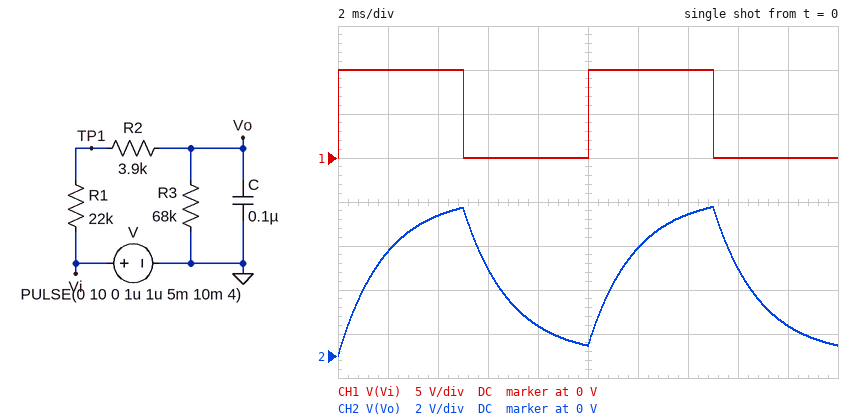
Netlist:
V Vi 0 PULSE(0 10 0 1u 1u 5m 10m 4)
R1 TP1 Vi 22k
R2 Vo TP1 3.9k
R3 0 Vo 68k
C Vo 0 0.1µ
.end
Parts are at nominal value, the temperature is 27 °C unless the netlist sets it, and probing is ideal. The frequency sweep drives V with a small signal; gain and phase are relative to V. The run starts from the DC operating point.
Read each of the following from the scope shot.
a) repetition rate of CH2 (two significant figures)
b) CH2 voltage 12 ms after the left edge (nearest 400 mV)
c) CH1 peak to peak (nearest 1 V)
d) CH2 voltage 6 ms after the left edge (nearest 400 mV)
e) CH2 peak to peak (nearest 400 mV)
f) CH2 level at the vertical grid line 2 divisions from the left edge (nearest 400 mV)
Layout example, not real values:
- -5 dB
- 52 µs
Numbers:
- 100 Hz
- 4.8 V
- 10 V
- 4.0 V
- 6.8 V
- 6.4 V
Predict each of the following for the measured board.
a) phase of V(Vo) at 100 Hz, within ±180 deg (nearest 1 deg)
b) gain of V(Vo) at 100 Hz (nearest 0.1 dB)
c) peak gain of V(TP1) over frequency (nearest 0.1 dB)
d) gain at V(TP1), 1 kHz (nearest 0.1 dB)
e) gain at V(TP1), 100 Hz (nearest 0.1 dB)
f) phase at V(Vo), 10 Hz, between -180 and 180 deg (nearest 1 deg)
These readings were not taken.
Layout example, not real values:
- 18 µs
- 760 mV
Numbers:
- -50 deg
- -6.6 dB
- -2.3 dB
- -15.7 dB
- -5.9 dB
- -7 deg
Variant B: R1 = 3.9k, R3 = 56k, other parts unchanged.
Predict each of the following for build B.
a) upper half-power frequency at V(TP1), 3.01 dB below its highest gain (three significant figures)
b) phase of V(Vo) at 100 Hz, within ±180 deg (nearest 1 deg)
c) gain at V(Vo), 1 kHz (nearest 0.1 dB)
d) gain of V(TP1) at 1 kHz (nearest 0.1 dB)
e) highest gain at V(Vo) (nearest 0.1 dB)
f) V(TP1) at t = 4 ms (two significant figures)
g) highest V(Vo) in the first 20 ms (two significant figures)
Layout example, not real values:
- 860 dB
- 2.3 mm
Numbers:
- 353 Hz
- -23 deg
- -14.0 dB
- -5.5 dB
- -1.1 dB
- 9.4 V
- 8.8 V
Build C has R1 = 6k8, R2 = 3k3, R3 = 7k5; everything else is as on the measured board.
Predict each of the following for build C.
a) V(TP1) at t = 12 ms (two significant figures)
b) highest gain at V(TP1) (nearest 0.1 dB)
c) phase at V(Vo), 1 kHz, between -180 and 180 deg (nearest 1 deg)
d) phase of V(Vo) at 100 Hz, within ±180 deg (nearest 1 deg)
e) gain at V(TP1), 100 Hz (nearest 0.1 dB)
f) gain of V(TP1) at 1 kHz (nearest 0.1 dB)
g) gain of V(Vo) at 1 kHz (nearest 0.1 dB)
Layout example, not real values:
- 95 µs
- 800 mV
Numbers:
- 6.1 V
- -4.2 dB
- -70 deg
- -15 deg
- -4.5 dB
- -8.6 dB
- -16.6 dB
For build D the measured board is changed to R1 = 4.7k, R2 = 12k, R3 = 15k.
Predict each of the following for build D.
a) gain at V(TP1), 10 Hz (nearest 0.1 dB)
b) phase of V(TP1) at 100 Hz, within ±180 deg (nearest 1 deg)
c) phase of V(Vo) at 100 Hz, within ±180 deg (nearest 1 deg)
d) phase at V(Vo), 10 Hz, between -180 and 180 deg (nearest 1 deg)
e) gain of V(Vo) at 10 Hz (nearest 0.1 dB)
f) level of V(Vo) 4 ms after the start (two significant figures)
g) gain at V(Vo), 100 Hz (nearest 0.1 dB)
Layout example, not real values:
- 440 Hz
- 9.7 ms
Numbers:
- -1.4 dB
- -4 deg
- -26 deg
- -3 deg
- -6.5 dB
- 4.7 V
- -7.5 dB
